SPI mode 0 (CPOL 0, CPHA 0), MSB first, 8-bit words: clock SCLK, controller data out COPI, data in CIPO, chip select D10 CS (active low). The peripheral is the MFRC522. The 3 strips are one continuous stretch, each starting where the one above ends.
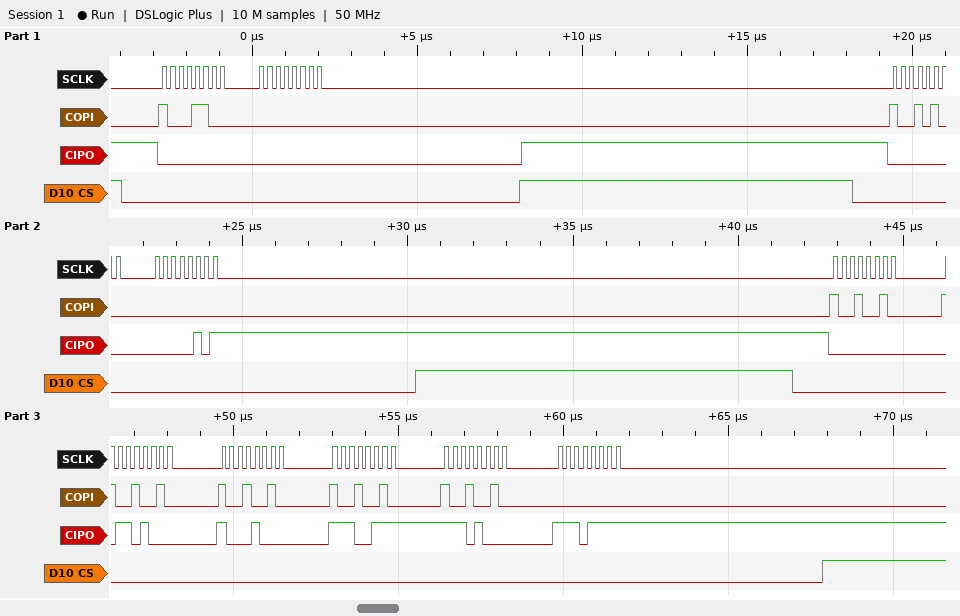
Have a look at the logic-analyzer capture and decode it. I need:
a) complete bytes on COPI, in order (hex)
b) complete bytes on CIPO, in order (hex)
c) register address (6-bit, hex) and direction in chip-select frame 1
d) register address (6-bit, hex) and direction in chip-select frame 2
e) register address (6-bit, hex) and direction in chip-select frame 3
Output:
8C 00 94 00 92 92 92 92 92 00
00 00 00 05 00 68 88 E7 E8 EF
0x06 read
0x0A read
0x09 read
